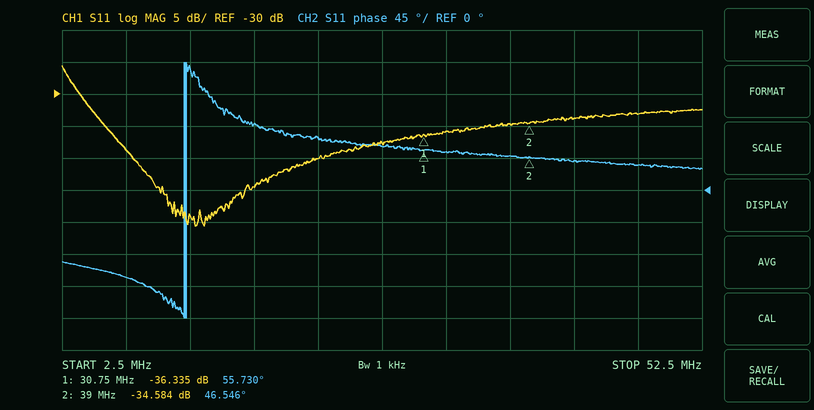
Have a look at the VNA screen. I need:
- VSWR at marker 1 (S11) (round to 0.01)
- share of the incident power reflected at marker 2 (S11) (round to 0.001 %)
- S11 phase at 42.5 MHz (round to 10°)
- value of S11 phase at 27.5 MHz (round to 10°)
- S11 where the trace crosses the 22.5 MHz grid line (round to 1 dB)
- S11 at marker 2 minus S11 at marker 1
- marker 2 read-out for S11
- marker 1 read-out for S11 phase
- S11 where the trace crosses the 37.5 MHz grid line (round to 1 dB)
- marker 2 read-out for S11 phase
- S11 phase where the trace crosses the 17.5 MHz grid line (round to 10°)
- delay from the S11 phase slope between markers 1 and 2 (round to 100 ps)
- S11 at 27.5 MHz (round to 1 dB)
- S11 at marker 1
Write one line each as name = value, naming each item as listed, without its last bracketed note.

VSWR at marker 1 (S11) = 1.03
share of the incident power reflected at marker 2 (S11) = 0.035 %
S11 phase at 42.5 MHz = 40°
value of S11 phase at 27.5 MHz = 60°
S11 where the trace crosses the 22.5 MHz grid line = -40 dB
S11 at marker 2 minus S11 at marker 1 = 1.751 dB
marker 2 read-out for S11 = -34.584 dB
marker 1 read-out for S11 phase = 55.730°
S11 where the trace crosses the 37.5 MHz grid line = -35 dB
marker 2 read-out for S11 phase = 46.546°
S11 phase where the trace crosses the 17.5 MHz grid line = 90°
delay from the S11 phase slope between markers 1 and 2 = 3.1 ns
S11 at 27.5 MHz = -38 dB
S11 at marker 1 = -36.335 dB
